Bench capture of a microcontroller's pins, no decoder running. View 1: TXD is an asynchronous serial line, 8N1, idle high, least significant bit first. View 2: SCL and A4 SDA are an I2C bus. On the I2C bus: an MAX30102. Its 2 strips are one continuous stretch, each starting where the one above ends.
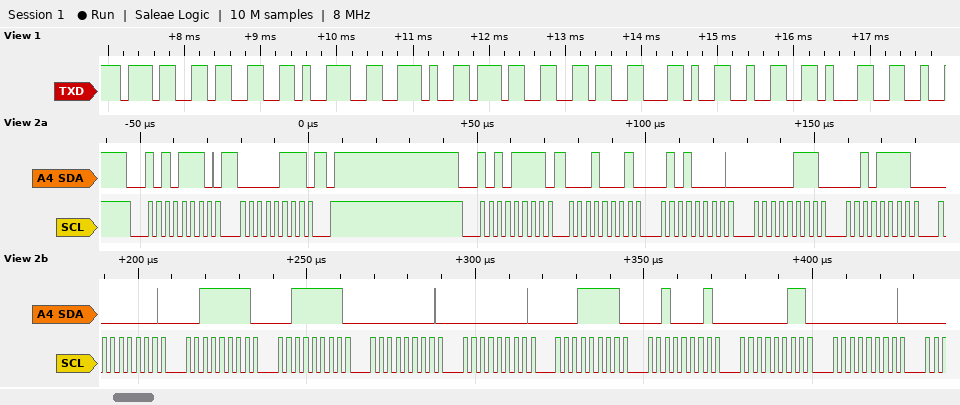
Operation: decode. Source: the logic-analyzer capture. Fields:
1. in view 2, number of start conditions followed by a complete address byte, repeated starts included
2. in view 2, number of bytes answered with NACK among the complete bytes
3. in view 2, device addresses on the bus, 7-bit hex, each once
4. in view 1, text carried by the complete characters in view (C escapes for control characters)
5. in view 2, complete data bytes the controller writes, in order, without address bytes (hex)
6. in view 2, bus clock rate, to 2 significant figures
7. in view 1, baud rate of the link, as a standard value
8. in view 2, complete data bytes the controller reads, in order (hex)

2
0
0x57
"739.76,21"
07
400 kHz
9600 baud
11 50 07 2F 00 3F 3F 00 00 1F 21 03 00
